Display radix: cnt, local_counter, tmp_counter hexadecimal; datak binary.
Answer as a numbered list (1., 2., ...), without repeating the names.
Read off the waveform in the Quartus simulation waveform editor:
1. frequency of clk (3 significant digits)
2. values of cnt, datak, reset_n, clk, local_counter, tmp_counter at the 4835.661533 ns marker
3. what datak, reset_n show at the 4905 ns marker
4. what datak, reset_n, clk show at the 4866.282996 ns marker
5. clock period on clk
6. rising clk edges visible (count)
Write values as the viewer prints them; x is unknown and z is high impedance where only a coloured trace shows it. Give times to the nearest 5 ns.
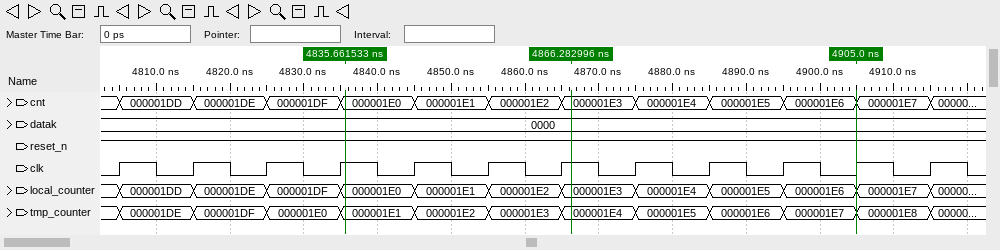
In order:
1. 100 MHz
2. cnt=000001E0, datak=0000, reset_n=1, clk=1, local_counter=000001E0, tmp_counter=000001E1
3. datak=0000, reset_n=1
4. datak=0000, reset_n=1, clk=1
5. 10 ns
6. 12
